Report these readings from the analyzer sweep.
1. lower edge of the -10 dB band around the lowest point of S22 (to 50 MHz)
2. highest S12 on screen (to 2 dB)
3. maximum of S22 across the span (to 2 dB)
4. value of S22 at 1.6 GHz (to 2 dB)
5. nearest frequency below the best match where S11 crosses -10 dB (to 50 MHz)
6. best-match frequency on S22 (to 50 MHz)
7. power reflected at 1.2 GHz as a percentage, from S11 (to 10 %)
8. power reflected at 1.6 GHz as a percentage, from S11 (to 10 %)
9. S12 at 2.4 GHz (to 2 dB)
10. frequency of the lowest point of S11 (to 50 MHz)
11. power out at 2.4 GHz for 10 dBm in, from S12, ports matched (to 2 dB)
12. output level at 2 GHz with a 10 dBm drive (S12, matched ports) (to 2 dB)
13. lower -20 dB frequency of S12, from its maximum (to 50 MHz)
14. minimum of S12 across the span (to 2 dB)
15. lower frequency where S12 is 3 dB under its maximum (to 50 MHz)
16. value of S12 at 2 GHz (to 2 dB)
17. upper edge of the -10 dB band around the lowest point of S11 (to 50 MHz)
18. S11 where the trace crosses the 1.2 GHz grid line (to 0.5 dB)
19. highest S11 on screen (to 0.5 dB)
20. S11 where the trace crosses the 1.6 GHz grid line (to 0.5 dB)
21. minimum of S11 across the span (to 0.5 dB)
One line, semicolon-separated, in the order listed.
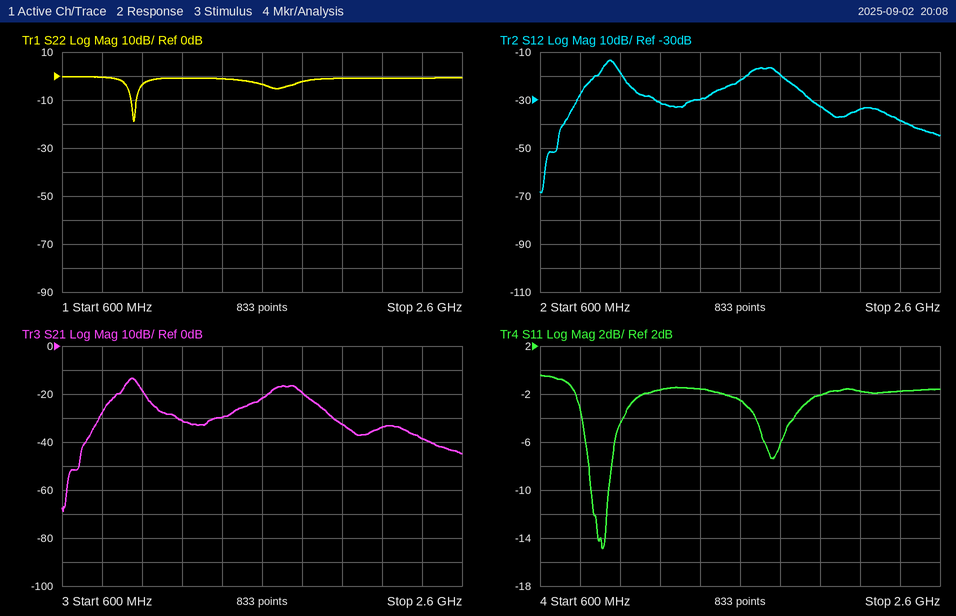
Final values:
950 MHz; -14 dB; 0 dB; -4 dB; 850 MHz; 950 MHz; 70 %; 60 %; -38 dB; 900 MHz; -28 dBm; -22 dBm; 750 MHz; -68 dB; 900 MHz; -32 dB; 950 MHz; -1.5 dB; -0.5 dB; -2.5 dB; -15.0 dB
